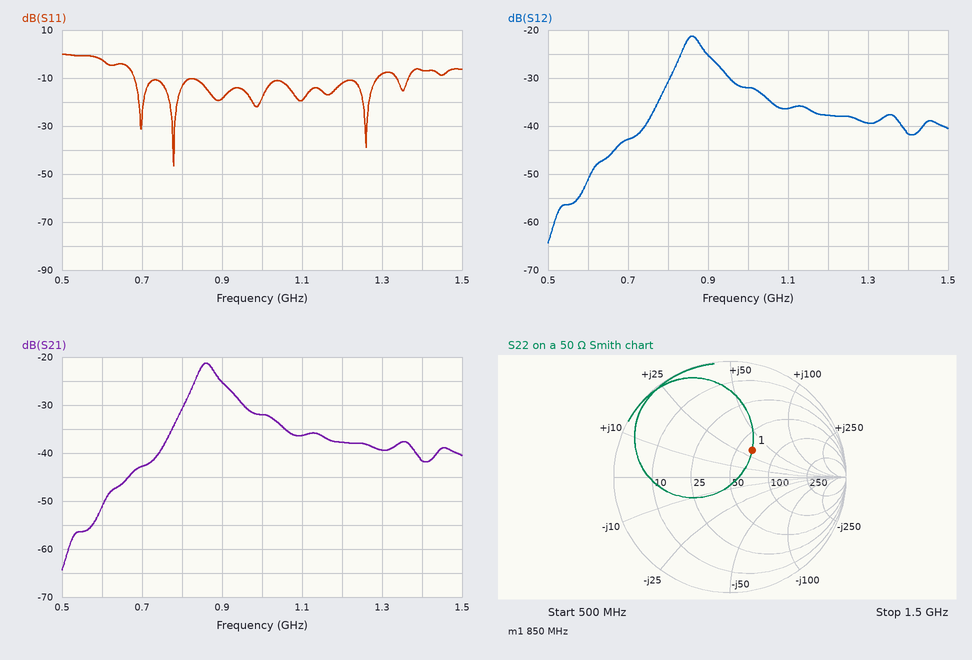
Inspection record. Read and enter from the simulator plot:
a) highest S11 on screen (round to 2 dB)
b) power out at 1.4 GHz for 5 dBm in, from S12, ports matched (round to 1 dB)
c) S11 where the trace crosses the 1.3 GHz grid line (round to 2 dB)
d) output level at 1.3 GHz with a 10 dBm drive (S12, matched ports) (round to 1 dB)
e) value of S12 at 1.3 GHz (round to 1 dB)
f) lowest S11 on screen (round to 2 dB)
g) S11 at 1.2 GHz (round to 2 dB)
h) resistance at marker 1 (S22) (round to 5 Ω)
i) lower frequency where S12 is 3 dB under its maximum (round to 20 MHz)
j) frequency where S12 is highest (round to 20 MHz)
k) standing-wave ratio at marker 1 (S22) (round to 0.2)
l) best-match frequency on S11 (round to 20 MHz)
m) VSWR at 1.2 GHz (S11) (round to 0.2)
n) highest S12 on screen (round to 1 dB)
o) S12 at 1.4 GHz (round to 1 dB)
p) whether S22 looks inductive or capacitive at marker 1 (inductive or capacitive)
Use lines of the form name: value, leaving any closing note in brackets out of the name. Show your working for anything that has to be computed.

highest S11 on screen: 0 dB
power out at 1.4 GHz for 5 dBm in, from S12, ports matched: 5 dBm + (-42 dB) = -37 dBm
S11 where the trace crosses the 1.3 GHz grid line: -8 dB
output level at 1.3 GHz with a 10 dBm drive (S12, matched ports): 10 dBm + (-39 dB) = -29 dBm
value of S12 at 1.3 GHz: -39 dB
lowest S11 on screen: -46 dB
S11 at 1.2 GHz: -12 dB
resistance at marker 1 (S22): 65 Ω
lower frequency where S12 is 3 dB under its maximum: 840 MHz
frequency where S12 is highest: 860 MHz
standing-wave ratio at marker 1 (S22): 1.8
best-match frequency on S11: 780 MHz
VSWR at 1.2 GHz (S11): |Γ| = 10^(-12/20) = 0.2512; VSWR = (1 + 0.2512)/(1 − 0.2512) ≈ 1.67, so 1.6 to the nearest 0.2
highest S12 on screen: -21 dB
S12 at 1.4 GHz: -42 dB
whether S22 looks inductive or capacitive at marker 1: inductive
